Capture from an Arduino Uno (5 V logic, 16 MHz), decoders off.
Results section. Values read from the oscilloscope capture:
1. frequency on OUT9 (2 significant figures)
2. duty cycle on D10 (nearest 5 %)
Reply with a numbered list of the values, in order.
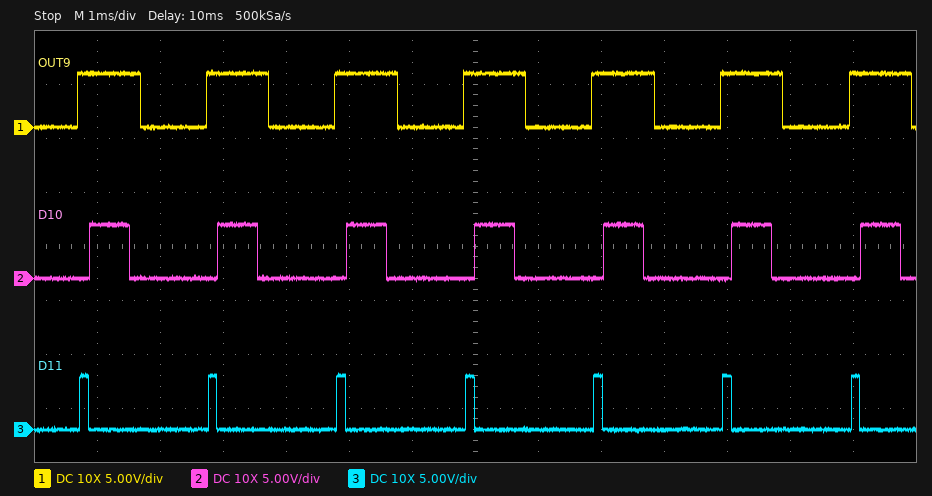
1. 490 Hz
2. 30 %
